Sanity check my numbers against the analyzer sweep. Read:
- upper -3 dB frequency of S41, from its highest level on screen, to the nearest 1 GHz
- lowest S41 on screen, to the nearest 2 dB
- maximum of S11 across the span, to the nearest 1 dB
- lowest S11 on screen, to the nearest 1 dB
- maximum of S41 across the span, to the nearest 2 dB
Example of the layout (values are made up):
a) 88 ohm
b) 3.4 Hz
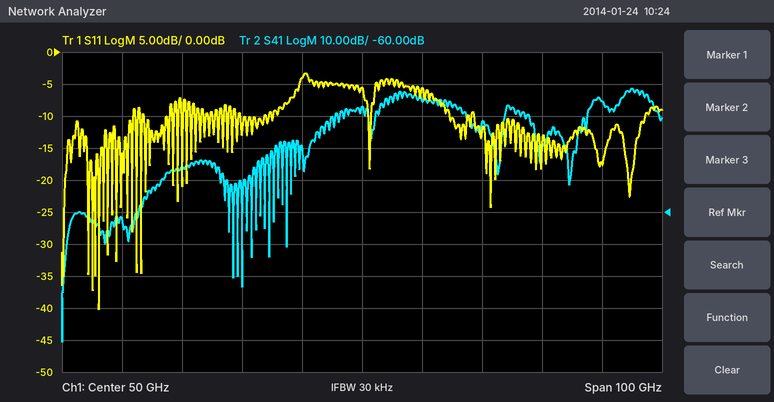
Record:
a) 98 GHz
b) -100 dB
c) -3 dB
d) -40 dB
e) -22 dB
